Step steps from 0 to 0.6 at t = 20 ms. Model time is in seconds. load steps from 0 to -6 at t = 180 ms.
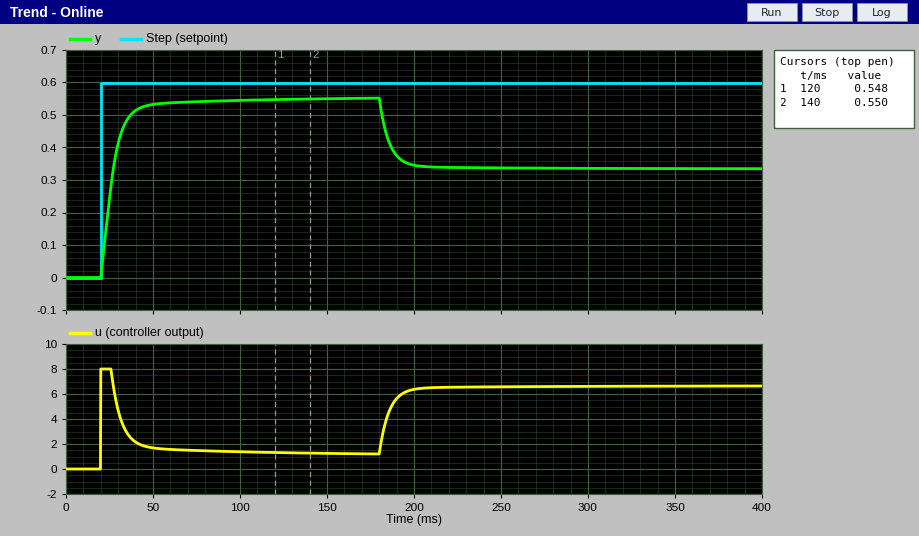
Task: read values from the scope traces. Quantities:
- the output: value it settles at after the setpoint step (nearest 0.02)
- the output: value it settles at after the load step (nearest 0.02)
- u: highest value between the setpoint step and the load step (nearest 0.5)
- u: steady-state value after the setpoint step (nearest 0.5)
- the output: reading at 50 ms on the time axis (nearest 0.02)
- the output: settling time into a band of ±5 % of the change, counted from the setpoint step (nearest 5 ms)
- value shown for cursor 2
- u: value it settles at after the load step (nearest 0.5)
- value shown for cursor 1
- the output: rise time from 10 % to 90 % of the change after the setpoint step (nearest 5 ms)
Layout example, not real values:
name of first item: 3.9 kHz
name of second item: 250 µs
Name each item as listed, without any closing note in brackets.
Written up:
the output: value it settles at after the setpoint step: 0.56
the output: value it settles at after the load step: 0.34
u: highest value between the setpoint step and the load step: 8.0
u: steady-state value after the setpoint step: 1.0
the output: reading at 50 ms on the time axis: 0.54
the output: settling time into a band of ±5 % of the change, counted from the setpoint step: 25 ms
value shown for cursor 2: 0.550
u: value it settles at after the load step: 6.5
value shown for cursor 1: 0.548
the output: rise time from 10 % to 90 % of the change after the setpoint step: 15 ms
